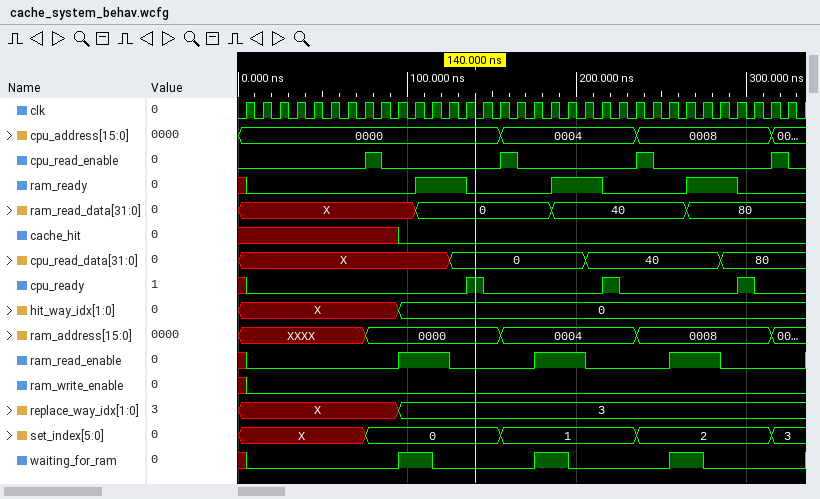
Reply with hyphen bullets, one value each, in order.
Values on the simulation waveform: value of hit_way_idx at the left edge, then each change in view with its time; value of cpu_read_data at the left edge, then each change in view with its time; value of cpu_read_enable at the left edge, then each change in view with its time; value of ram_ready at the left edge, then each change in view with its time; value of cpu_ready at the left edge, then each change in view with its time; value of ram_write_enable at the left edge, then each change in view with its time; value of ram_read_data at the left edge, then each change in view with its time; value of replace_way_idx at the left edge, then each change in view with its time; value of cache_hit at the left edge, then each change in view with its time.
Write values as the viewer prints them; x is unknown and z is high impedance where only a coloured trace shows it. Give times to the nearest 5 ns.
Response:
- X, 0 at 95 ns
- X, 0 at 125 ns, 40 at 205 ns, 80 at 285 ns
- 0, 1 at 75 ns, 0 at 85 ns, 1 at 155 ns, 0 at 165 ns, 1 at 235 ns, 0 at 245 ns, 1 at 315 ns, 0 at 325 ns
- x, 0 at 5 ns, 1 at 105 ns, 0 at 135 ns, 1 at 185 ns, 0 at 215 ns, 1 at 265 ns, 0 at 295 ns
- x, 0 at 5 ns, 1 at 135 ns, 0 at 145 ns, 1 at 215 ns, 0 at 225 ns, 1 at 295 ns, 0 at 305 ns
- x, 0 at 5 ns
- X, 0 at 105 ns, 40 at 185 ns, 80 at 265 ns
- X, 3 at 95 ns
- x, 0 at 95 ns
